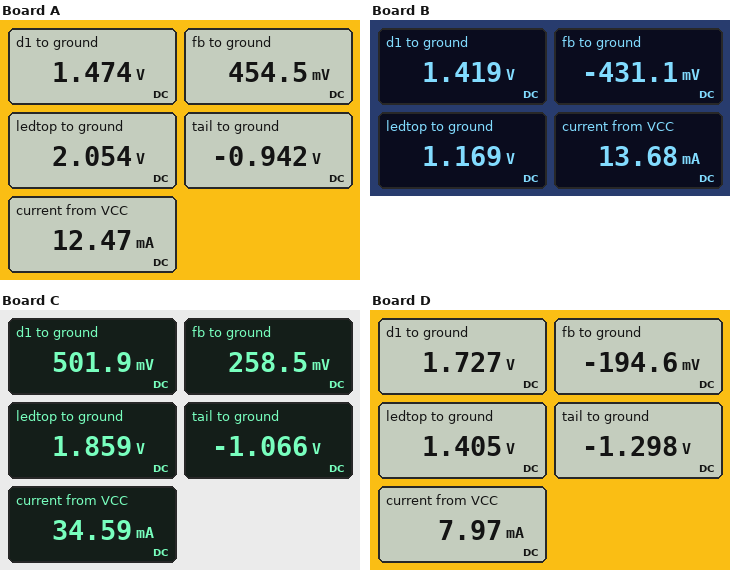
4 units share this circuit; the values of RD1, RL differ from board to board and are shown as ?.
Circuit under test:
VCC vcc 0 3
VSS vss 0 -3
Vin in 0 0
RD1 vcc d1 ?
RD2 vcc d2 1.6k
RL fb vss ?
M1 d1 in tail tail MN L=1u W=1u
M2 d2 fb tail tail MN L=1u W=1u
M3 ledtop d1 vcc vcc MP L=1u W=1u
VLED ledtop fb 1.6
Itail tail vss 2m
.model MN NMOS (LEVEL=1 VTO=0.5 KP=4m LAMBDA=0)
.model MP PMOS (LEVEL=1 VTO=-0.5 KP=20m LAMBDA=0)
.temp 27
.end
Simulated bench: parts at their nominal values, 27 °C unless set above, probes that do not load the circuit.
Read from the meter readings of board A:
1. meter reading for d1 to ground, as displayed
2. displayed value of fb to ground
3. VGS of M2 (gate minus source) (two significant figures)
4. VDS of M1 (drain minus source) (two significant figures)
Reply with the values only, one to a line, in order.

1.474 V
454.5 mV
1.4 V
2.4 V
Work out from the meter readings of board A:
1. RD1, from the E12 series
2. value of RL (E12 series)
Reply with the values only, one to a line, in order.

3.9 kΩ
330 Ω
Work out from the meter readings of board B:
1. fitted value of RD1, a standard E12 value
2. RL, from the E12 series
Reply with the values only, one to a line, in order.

1 kΩ
220 Ω
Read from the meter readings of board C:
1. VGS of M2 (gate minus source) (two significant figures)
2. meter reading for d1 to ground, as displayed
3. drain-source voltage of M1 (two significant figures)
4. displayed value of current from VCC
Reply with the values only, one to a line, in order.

1.3 V
501.9 mV
1.6 V
34.59 mA
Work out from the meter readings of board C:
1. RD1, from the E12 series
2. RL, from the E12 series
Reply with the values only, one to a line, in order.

3.9 kΩ
100 Ω
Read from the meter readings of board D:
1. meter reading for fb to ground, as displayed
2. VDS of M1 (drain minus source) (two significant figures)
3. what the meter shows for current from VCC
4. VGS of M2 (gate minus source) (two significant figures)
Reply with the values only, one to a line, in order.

-194.6 mV
3.0 V
7.97 mA
1.1 V
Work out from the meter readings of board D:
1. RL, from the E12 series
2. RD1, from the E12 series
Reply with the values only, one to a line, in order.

470 Ω
1 kΩ
